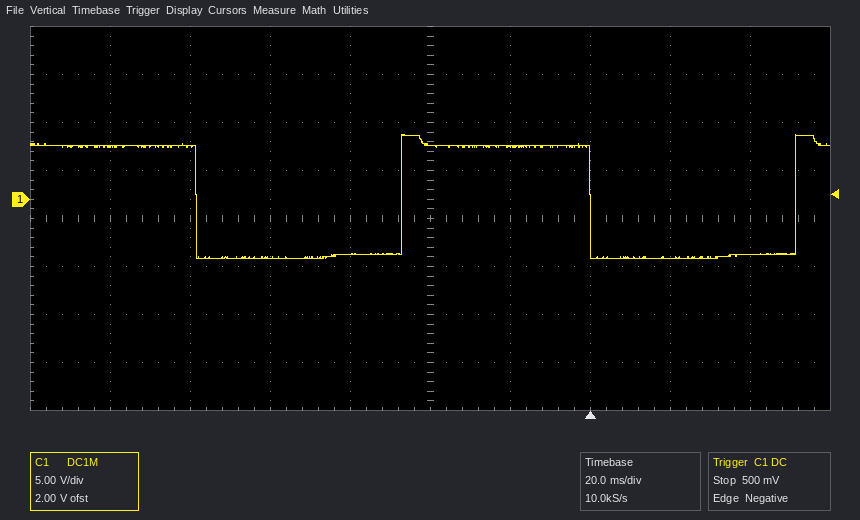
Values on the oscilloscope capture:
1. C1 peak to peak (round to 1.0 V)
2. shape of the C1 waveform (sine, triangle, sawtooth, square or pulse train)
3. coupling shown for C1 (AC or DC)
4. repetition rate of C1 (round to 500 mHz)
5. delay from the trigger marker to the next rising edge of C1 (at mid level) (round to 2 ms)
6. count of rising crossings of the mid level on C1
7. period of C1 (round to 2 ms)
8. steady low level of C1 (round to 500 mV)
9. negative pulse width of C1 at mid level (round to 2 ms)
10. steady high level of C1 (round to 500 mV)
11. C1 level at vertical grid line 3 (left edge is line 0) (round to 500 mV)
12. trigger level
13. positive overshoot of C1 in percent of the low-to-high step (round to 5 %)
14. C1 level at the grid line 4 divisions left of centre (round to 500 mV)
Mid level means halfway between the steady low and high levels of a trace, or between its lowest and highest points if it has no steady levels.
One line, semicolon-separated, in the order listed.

13.0 V; square; DC; 10.0 Hz; 52 ms; 2; 98 ms; -6.0 V; 52 ms; 5.5 V; -6.0 V; 500 mV; 10 %; 5.5 V
